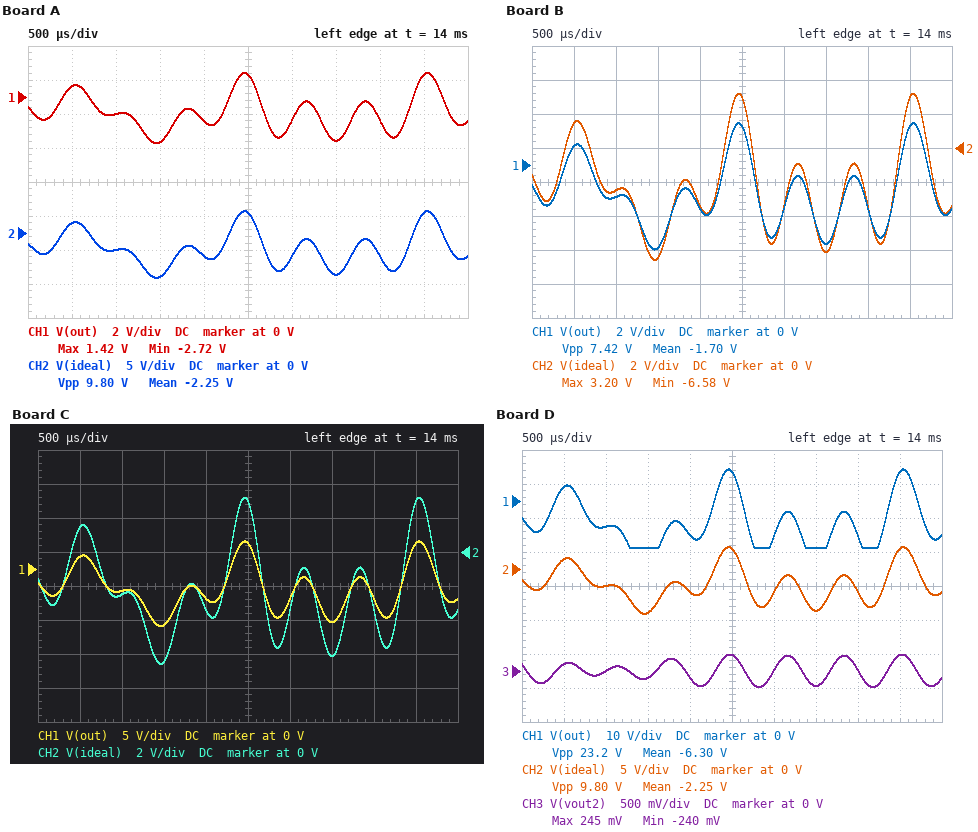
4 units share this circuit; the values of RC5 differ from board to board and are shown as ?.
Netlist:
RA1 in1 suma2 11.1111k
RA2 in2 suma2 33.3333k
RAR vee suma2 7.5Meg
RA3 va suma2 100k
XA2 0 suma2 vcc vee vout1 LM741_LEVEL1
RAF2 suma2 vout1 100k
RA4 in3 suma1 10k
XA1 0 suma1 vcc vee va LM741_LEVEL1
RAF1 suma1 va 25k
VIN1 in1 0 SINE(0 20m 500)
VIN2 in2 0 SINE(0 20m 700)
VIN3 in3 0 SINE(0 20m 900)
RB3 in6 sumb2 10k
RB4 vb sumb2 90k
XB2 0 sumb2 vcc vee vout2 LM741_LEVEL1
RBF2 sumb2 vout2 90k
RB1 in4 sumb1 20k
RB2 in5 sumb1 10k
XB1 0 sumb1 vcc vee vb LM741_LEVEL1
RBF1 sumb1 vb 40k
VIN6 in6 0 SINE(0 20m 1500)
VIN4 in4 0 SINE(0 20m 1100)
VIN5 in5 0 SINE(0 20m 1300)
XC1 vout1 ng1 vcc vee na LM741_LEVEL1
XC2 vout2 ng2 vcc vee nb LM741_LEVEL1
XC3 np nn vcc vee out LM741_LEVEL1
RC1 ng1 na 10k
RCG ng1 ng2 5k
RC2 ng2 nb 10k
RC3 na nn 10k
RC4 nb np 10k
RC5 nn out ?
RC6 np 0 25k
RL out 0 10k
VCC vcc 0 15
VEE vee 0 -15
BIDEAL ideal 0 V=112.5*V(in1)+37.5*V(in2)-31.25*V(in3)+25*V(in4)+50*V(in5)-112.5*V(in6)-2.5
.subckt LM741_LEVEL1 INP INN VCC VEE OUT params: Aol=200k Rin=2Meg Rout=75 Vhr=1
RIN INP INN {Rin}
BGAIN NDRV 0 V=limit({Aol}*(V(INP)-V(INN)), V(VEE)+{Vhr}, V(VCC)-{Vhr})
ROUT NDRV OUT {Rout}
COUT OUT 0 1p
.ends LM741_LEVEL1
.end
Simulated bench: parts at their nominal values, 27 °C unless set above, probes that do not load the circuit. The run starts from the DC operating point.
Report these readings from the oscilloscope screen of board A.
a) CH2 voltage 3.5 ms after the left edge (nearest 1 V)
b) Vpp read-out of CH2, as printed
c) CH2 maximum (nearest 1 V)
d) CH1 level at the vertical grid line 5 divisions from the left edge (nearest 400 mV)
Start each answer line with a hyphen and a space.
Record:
- -6 V
- 9.80 V
- 3 V
- 1.2 V
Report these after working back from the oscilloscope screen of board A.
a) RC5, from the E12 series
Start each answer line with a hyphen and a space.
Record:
- 8.2 kΩ
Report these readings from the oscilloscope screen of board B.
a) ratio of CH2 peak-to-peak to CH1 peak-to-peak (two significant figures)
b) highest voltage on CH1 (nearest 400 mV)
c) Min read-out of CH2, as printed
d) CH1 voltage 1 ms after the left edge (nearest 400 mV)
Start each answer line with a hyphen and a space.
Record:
- 1.3
- 2.4 V
- -6.58 V
- -2.0 V
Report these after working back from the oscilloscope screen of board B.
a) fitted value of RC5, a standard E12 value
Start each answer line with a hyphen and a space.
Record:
- 18 kΩ
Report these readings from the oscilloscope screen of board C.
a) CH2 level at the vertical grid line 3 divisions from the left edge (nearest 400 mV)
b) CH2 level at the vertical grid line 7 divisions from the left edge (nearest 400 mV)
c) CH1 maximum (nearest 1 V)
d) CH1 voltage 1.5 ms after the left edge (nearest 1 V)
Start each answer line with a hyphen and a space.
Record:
- -6.4 V
- -6.0 V
- 4 V
- -8 V
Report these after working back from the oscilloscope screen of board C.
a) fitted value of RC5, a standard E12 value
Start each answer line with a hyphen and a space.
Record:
- 33 kΩ
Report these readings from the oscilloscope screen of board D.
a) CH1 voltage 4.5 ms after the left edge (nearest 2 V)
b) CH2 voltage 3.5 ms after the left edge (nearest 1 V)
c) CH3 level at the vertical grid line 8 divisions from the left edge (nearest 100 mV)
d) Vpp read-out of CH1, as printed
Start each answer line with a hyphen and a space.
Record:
- 8 V
- -6 V
- 0 V
- 23.2 V
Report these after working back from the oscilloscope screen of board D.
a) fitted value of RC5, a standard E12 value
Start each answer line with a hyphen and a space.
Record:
- 82 kΩ
